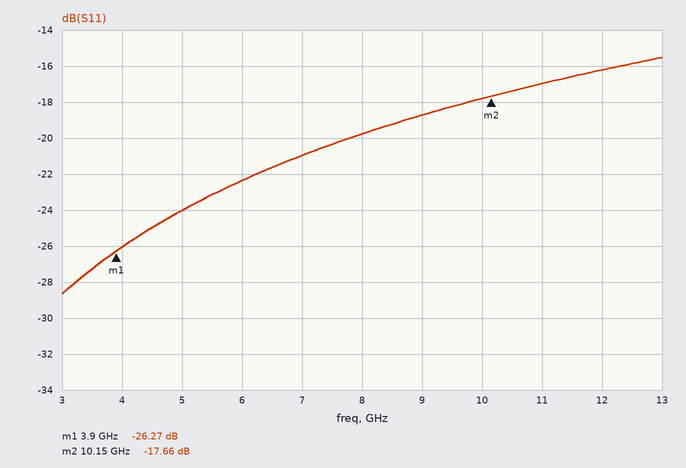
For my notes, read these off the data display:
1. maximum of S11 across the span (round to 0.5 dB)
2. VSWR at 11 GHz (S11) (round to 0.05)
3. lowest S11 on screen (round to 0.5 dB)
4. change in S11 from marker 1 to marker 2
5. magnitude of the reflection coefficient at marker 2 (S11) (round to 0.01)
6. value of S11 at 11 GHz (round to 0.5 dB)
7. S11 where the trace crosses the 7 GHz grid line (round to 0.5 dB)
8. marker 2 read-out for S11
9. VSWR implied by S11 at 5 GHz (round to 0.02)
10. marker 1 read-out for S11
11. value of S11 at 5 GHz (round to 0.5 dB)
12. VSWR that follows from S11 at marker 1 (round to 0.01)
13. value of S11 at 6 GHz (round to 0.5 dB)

-15.5 dB
1.35
-28.5 dB
8.61 dB
0.13
-17.0 dB
-21.0 dB
-17.66 dB
1.14
-26.27 dB
-24.0 dB
1.10
-22.5 dB
